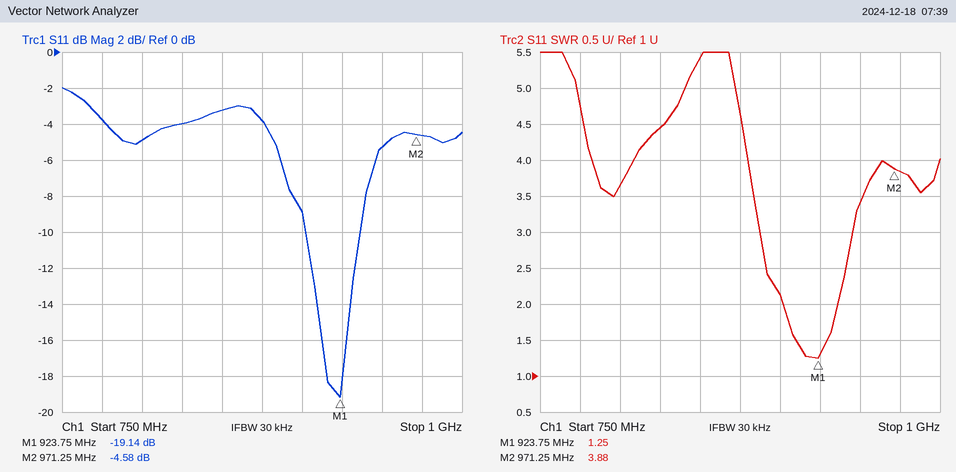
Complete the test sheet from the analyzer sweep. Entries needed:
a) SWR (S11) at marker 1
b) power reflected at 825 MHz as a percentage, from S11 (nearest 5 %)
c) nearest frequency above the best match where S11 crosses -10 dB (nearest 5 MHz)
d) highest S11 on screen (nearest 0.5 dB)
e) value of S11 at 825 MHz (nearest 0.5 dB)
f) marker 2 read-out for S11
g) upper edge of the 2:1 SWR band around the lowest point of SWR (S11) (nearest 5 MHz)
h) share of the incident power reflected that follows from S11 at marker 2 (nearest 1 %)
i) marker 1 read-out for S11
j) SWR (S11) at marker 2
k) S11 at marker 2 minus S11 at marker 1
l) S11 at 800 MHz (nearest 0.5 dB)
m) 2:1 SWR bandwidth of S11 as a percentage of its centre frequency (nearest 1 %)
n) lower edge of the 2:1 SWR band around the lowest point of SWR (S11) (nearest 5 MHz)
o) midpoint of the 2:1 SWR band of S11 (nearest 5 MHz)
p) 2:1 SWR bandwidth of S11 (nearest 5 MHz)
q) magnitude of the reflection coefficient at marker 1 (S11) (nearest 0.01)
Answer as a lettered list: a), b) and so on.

a) 1.25
b) 40 %
c) 935 MHz
d) -2.0 dB
e) -4.0 dB
f) -4.58 dB
g) 935 MHz
h) 35 %
i) -19.14 dB
j) 3.88
k) 14.56 dB
l) -5.0 dB
m) 4 %
n) 900 MHz
o) 920 MHz
p) 35 MHz
q) 0.11
